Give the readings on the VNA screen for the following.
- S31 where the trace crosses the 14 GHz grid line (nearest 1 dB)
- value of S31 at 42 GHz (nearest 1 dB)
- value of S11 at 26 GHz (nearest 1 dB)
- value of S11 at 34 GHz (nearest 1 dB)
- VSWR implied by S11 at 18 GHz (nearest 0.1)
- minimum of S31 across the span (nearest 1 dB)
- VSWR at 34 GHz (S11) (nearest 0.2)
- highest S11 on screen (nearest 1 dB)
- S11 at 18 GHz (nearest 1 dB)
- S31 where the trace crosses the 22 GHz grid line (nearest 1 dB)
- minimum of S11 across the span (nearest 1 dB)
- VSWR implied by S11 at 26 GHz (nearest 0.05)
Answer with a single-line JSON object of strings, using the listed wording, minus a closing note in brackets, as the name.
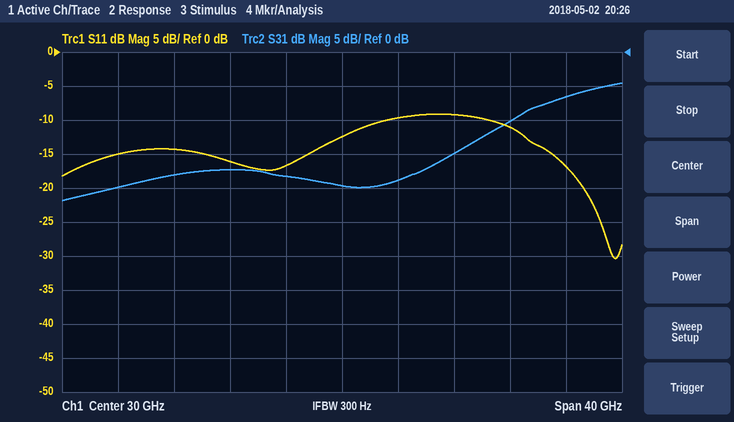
{"S31 where the trace crosses the 14 GHz grid line": "-20 dB", "value of S31 at 42 GHz": "-10 dB", "value of S11 at 26 GHz": "-17 dB", "value of S11 at 34 GHz": "-10 dB", "VSWR implied by S11 at 18 GHz": "1.5", "minimum of S31 across the span": "-22 dB", "VSWR at 34 GHz (S11)": "2.0", "highest S11 on screen": "-9 dB", "S11 at 18 GHz": "-14 dB", "S31 where the trace crosses the 22 GHz grid line": "-17 dB", "minimum of S11 across the span": "-30 dB", "VSWR implied by S11 at 26 GHz": "1.35"}
